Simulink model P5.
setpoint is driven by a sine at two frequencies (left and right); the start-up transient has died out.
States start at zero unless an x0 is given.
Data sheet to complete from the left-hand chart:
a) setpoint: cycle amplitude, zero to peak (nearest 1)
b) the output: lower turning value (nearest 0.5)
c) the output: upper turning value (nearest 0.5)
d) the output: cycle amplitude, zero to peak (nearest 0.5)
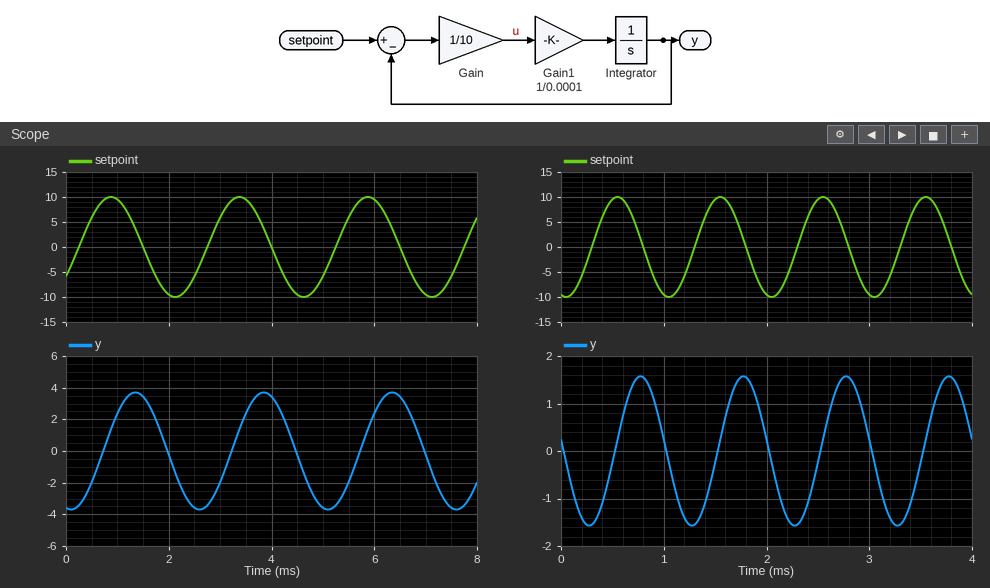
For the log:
10
-3.5
3.5
3.5
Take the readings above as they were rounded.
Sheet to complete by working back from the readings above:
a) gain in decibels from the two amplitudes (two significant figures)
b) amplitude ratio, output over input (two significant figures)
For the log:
-9.1 dB
0.35
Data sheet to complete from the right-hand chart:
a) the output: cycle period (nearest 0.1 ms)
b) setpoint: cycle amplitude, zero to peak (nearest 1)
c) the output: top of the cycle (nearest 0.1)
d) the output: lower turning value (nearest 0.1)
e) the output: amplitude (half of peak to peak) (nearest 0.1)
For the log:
1.0 ms
10
1.6
-1.6
1.6
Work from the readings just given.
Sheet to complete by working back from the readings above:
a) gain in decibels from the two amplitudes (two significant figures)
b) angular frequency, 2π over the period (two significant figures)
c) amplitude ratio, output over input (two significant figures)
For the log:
-16 dB
6.3 rad/ms
0.16
